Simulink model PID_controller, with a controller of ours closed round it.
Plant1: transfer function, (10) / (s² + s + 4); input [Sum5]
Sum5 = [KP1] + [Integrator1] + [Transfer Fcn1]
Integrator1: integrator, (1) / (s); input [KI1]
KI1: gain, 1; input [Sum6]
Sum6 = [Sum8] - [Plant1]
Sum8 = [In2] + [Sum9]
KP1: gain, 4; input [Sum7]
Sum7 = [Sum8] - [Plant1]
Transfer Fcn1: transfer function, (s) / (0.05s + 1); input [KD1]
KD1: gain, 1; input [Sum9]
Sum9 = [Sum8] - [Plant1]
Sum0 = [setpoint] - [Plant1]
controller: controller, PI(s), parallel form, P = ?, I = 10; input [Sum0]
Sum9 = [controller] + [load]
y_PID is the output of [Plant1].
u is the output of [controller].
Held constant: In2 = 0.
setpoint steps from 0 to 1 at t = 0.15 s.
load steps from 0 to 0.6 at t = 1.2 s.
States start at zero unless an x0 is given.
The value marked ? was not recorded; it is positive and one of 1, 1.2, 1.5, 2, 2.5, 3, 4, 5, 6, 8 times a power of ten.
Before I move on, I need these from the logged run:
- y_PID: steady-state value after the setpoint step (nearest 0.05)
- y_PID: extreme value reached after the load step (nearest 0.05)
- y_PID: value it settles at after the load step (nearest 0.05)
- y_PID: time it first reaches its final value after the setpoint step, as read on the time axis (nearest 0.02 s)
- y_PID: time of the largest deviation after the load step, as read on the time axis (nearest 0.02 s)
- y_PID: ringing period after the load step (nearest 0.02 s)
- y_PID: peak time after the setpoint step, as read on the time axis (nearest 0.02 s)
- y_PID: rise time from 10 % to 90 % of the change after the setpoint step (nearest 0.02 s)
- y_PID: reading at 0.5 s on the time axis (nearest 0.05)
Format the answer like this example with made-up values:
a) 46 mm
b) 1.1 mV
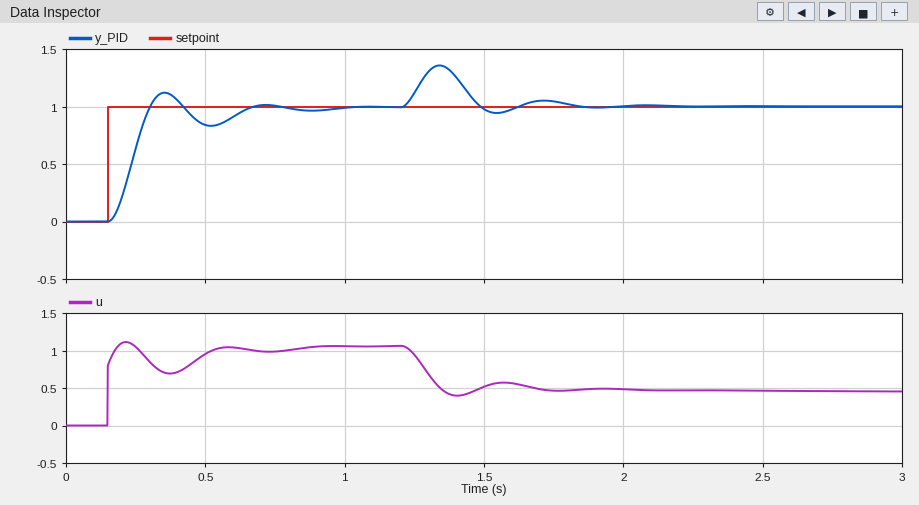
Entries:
a) 1.00
b) 1.35
c) 1.00
d) 0.30 s
e) 1.34 s
f) 0.38 s
g) 0.36 s
h) 0.10 s
i) 0.85
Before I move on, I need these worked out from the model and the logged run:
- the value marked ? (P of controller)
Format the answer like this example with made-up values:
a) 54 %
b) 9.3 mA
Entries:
a) 0.8
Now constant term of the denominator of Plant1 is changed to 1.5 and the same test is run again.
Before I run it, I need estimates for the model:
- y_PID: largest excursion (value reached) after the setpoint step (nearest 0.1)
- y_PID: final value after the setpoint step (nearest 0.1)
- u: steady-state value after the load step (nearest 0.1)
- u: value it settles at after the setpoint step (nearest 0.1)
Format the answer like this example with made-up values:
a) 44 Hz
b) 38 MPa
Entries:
a) 1.1
b) 1.0
c) 0.4
d) 1.0
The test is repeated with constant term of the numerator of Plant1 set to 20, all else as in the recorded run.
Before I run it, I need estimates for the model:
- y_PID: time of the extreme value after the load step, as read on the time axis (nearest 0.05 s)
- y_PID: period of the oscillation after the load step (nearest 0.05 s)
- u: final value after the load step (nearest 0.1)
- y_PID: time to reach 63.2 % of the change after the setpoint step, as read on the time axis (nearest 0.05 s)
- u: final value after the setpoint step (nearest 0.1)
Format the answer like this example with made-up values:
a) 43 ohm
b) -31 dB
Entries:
a) 1.30 s
b) 0.25 s
c) 0.4
d) 0.20 s
e) 1.0
